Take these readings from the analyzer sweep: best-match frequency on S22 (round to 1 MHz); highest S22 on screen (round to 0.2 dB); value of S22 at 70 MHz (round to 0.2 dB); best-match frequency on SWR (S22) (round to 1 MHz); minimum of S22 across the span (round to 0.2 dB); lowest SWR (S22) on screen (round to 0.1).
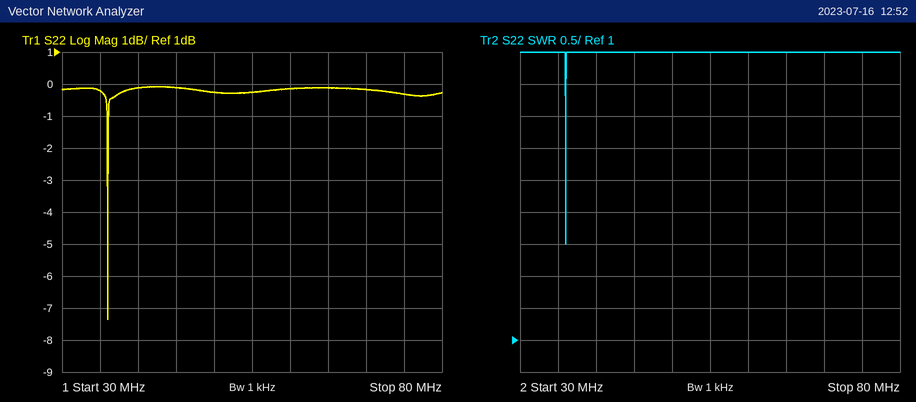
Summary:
36 MHz
0.0 dB
-0.2 dB
36 MHz
-7.4 dB
2.5
